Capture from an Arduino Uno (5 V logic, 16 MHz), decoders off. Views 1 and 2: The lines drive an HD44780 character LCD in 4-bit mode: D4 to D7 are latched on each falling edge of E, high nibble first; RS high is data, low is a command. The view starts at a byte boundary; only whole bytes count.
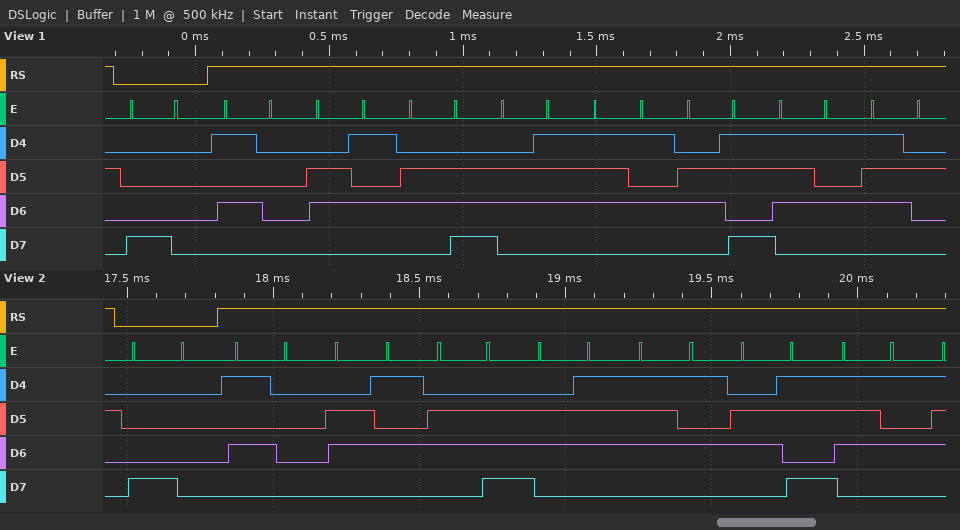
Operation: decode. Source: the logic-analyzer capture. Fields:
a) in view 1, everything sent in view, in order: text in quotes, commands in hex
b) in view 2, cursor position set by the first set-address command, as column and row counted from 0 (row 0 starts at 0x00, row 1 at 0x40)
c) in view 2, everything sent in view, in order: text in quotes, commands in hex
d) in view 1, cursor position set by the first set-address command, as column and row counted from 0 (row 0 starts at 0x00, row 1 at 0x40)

0x80 "Pengukur"
column 0, row 0
0x80 "Penguku"
column 0, row 0
